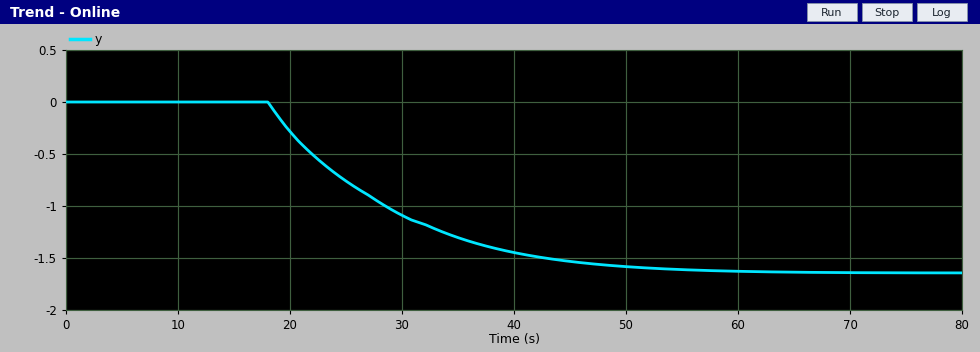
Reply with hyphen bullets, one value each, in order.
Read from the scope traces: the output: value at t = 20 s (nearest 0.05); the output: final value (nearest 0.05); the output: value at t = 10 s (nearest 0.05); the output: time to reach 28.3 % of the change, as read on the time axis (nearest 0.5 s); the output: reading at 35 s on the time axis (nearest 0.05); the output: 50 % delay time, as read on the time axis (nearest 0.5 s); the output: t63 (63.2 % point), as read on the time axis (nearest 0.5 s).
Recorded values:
- -0.30
- -1.65
- 0.00
- 21.5 s
- -1.30
- 26.0 s
- 29.0 s
